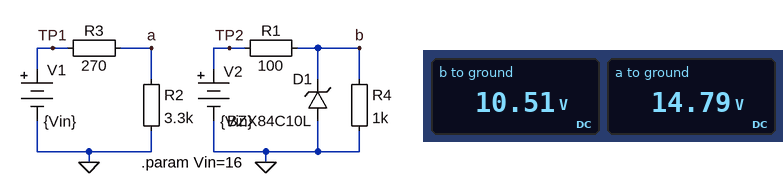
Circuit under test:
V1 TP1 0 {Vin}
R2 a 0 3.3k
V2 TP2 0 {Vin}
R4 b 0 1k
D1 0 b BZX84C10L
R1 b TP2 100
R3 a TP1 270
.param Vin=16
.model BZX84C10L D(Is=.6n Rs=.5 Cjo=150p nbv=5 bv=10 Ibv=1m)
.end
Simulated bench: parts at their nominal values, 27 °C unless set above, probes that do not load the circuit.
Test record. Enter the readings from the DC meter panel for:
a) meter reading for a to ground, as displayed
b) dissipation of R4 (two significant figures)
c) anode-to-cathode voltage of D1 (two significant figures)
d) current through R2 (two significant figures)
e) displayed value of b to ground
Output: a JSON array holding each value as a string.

["14.79 V", "110 mW", "-11 V", "4.5 mA", "10.51 V"]
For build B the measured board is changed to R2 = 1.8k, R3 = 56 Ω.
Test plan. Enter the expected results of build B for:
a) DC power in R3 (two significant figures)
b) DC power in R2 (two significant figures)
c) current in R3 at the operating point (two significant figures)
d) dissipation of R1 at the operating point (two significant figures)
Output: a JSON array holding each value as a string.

["4.2 mW", "130 mW", "8.6 mA", "300 mW"]
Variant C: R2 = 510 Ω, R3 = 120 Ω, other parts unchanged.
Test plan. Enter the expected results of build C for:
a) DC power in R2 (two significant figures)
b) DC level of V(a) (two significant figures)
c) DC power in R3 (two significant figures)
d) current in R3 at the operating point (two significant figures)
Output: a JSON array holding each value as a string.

["330 mW", "13 V", "77 mW", "25 mA"]
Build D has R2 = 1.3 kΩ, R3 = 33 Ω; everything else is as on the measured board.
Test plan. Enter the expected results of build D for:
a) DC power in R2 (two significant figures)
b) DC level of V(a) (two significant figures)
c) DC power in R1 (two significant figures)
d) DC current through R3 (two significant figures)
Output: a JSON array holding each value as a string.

["190 mW", "16 V", "300 mW", "12 mA"]
